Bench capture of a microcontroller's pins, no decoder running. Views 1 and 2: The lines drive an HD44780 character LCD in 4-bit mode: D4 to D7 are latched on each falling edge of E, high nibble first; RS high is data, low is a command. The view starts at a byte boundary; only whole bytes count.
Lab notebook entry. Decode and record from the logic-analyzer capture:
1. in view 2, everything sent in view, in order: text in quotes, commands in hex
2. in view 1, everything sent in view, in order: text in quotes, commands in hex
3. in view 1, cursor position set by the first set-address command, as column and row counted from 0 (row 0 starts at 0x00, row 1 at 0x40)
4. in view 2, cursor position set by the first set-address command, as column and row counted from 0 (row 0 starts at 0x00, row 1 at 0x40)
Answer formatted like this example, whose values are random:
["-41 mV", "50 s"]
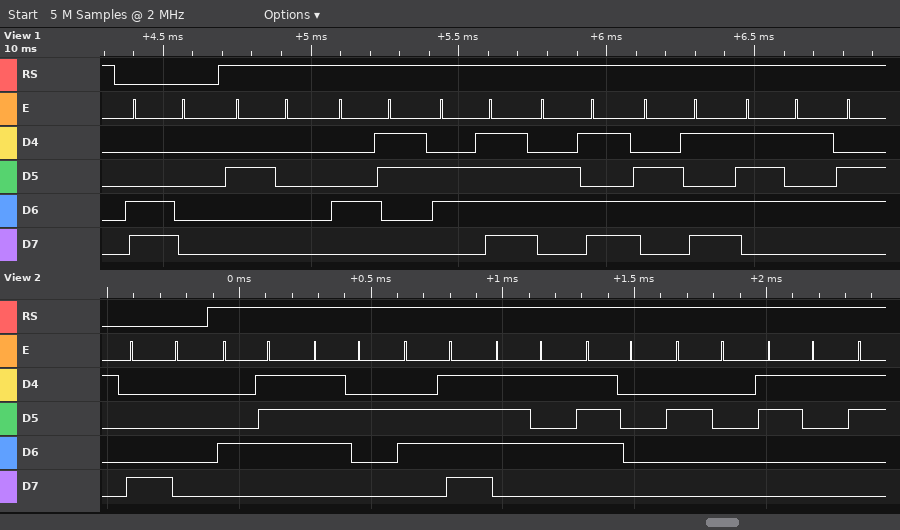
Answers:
["0x80 \"Group 1\"", "0xC0 \" Commu\"", "column 0, row 1", "column 0, row 0"]
